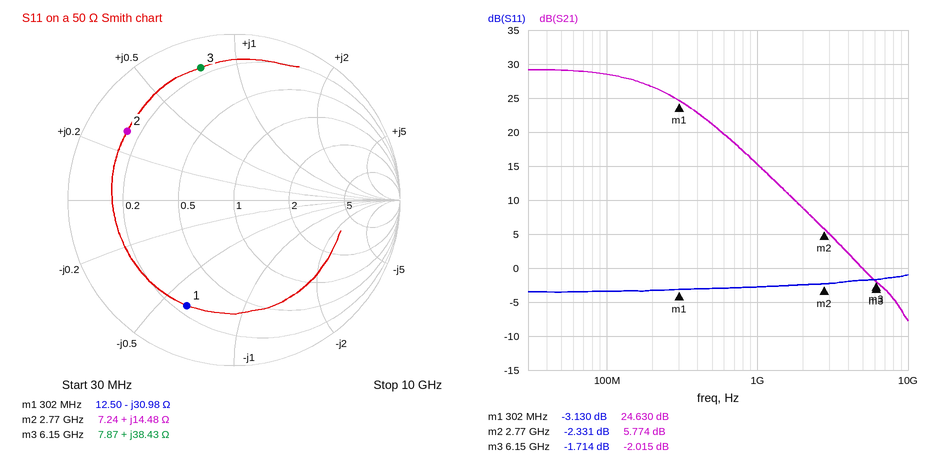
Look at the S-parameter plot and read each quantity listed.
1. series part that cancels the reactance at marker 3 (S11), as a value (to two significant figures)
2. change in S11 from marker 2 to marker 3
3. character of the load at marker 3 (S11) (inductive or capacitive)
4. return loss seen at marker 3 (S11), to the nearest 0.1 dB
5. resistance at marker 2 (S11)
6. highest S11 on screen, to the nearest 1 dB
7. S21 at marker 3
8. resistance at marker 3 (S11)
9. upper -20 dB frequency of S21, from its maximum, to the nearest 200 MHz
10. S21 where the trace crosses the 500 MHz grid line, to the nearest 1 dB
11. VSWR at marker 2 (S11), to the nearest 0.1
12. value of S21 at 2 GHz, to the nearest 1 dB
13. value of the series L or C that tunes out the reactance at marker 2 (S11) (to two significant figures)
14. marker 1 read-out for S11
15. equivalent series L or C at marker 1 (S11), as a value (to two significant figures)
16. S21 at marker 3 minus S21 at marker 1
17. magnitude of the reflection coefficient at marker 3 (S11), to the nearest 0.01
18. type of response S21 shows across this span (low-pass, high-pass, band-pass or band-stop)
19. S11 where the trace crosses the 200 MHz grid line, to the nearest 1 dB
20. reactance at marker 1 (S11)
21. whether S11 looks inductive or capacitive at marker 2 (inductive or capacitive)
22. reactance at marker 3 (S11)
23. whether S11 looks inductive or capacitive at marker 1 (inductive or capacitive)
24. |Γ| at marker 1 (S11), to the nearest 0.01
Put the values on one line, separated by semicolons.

670 fF; 0.617 dB; inductive; 1.7 dB; 7.24 Ω; -1 dB; -2.015 dB; 7.87 Ω; 2.0 GHz; 21 dB; 7.5; 9 dB; 4.0 pF; -3.130 dB; 17 pF; -26.645 dB; 0.82; low-pass; -3 dB; -30.98 Ω; inductive; +38.43 Ω; capacitive; 0.70
